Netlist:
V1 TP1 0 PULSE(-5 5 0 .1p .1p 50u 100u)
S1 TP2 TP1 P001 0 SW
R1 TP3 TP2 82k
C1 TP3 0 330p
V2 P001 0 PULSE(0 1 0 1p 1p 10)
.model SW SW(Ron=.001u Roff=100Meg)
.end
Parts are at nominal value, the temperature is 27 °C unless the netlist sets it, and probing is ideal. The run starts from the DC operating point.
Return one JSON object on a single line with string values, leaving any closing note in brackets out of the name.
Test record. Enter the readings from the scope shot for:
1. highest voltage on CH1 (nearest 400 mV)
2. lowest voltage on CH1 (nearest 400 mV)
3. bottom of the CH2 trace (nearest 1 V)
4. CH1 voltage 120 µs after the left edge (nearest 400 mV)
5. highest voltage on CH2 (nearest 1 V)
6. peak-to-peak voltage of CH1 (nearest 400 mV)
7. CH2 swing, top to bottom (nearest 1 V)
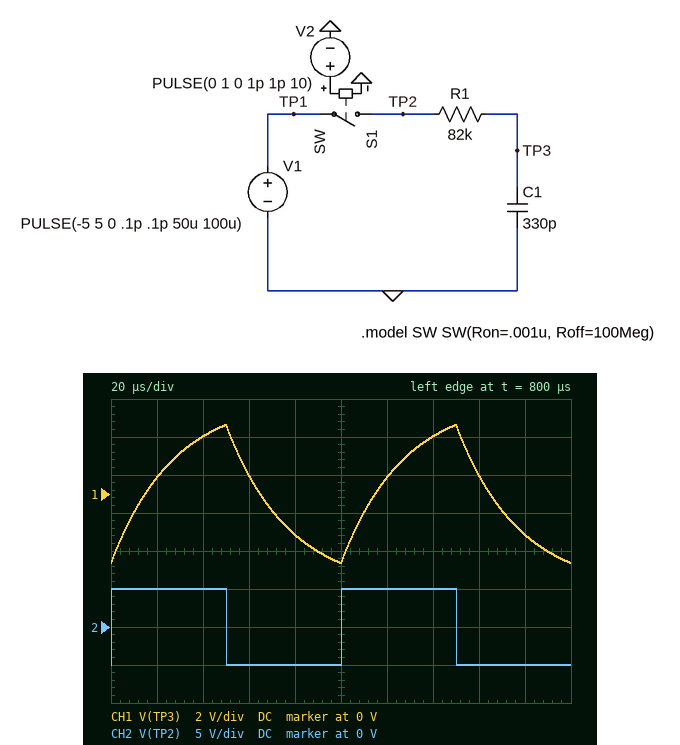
{"highest voltage on CH1": "3.6 V", "lowest voltage on CH1": "-3.6 V", "bottom of the CH2 trace": "-5 V", "CH1 voltage 120 µs after the left edge": "800 mV", "highest voltage on CH2": "5 V", "peak-to-peak voltage of CH1": "7.2 V", "CH2 swing, top to bottom": "10 V"}
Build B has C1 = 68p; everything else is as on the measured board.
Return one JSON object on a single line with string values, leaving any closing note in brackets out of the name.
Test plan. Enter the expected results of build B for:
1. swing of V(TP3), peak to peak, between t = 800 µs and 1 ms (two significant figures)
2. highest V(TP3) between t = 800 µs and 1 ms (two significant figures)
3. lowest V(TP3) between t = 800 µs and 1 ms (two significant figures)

{"swing of V(TP3), peak to peak, between t = 800 µs and 1 ms": "10 V", "highest V(TP3) between t = 800 µs and 1 ms": "5.0 V", "lowest V(TP3) between t = 800 µs and 1 ms": "-5.0 V"}
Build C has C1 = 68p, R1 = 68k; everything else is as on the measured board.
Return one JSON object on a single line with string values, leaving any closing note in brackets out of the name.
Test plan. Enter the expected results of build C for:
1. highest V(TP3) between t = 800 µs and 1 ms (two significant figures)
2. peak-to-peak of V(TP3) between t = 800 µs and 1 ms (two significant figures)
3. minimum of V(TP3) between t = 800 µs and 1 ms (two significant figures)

{"highest V(TP3) between t = 800 µs and 1 ms": "5.0 V", "peak-to-peak of V(TP3) between t = 800 µs and 1 ms": "10 V", "minimum of V(TP3) between t = 800 µs and 1 ms": "-5.0 V"}
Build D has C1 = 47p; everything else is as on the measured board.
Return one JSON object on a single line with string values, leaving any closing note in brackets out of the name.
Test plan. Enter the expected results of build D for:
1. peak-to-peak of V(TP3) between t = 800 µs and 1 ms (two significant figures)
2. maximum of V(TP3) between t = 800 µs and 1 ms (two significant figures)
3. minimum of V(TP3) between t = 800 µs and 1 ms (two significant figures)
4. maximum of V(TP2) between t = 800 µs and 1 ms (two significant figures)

{"peak-to-peak of V(TP3) between t = 800 µs and 1 ms": "10 V", "maximum of V(TP3) between t = 800 µs and 1 ms": "5.0 V", "minimum of V(TP3) between t = 800 µs and 1 ms": "-5.0 V", "maximum of V(TP2) between t = 800 µs and 1 ms": "5.0 V"}
